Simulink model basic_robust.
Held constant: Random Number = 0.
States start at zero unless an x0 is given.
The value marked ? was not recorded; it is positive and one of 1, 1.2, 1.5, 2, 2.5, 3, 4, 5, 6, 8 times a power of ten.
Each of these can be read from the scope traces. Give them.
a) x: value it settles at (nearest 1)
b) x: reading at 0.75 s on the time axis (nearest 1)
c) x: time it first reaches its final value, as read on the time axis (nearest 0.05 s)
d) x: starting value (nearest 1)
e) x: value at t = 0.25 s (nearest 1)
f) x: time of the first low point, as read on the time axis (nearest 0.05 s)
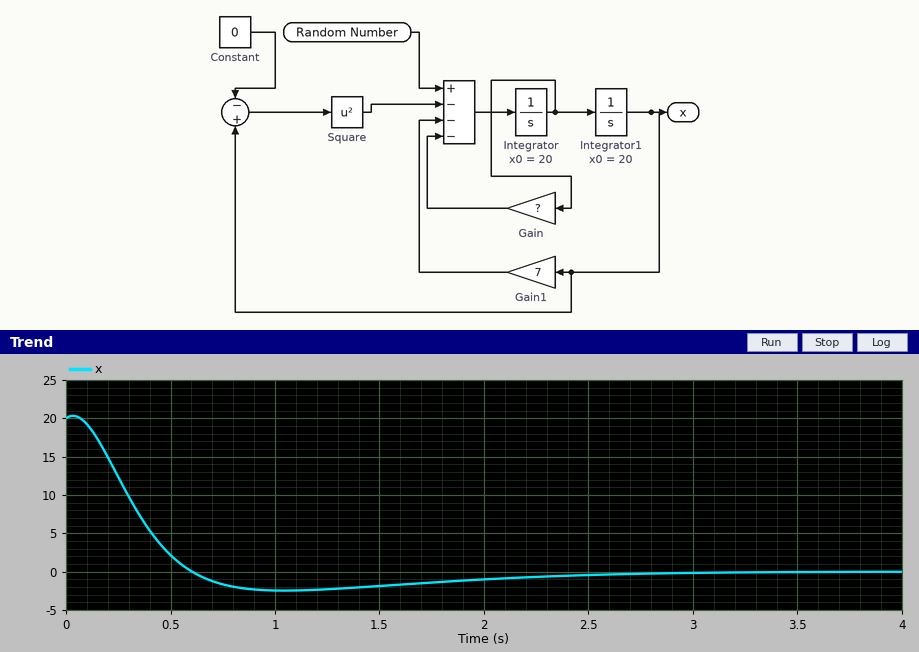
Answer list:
0
-2
0.60 s
20
12
1.05 s
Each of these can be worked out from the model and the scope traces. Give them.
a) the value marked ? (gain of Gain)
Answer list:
5
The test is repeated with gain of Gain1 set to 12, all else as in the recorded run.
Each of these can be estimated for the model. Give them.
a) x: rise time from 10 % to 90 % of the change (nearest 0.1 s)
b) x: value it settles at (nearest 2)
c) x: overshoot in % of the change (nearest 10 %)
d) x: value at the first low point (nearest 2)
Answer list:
0.3 s
0
20 %
-4
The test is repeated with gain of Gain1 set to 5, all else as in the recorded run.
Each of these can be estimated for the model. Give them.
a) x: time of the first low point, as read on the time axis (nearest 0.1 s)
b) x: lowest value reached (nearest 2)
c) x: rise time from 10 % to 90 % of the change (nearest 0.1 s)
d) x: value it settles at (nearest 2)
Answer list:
1.2 s
-2
0.4 s
0
